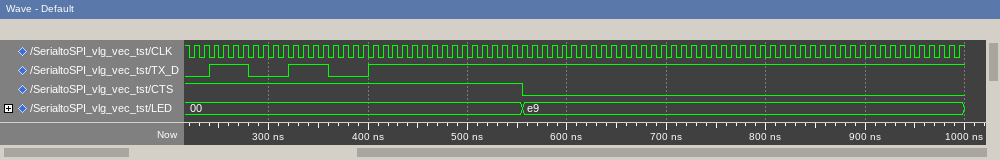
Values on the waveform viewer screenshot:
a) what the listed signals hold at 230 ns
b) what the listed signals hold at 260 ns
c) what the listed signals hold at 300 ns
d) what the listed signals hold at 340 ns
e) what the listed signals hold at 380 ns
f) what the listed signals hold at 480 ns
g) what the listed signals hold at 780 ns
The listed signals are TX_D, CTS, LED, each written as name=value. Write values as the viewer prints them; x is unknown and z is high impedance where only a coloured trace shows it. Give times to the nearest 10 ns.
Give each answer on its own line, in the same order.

TX_D=0, CTS=1, LED=00
TX_D=1, CTS=1, LED=00
TX_D=0, CTS=1, LED=00
TX_D=1, CTS=1, LED=00
TX_D=0, CTS=1, LED=00
TX_D=1, CTS=1, LED=00
TX_D=1, CTS=0, LED=e9
